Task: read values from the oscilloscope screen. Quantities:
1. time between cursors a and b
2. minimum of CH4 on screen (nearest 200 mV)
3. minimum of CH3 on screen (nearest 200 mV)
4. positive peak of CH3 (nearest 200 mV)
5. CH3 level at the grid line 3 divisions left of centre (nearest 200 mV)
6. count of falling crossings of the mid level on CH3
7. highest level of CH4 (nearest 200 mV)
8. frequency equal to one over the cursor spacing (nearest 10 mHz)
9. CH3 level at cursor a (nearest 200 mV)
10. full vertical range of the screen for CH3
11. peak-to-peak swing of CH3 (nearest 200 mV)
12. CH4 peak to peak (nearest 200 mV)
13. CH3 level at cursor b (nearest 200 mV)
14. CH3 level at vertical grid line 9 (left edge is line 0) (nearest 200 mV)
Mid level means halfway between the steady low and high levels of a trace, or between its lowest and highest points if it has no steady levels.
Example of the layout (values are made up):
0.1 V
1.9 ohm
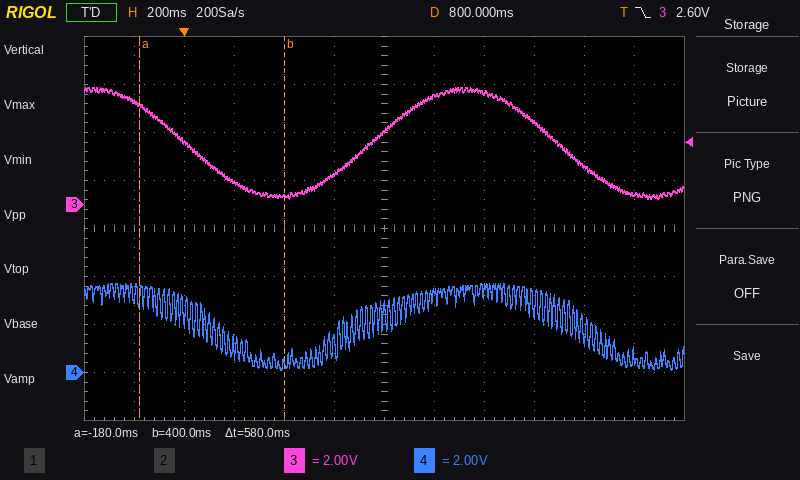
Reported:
580 ms
200 mV
200 mV
4.8 V
1.0 V
2
3.8 V
1.72 Hz
4.2 V
16 V
4.6 V
3.6 V
400 mV
3.4 V
